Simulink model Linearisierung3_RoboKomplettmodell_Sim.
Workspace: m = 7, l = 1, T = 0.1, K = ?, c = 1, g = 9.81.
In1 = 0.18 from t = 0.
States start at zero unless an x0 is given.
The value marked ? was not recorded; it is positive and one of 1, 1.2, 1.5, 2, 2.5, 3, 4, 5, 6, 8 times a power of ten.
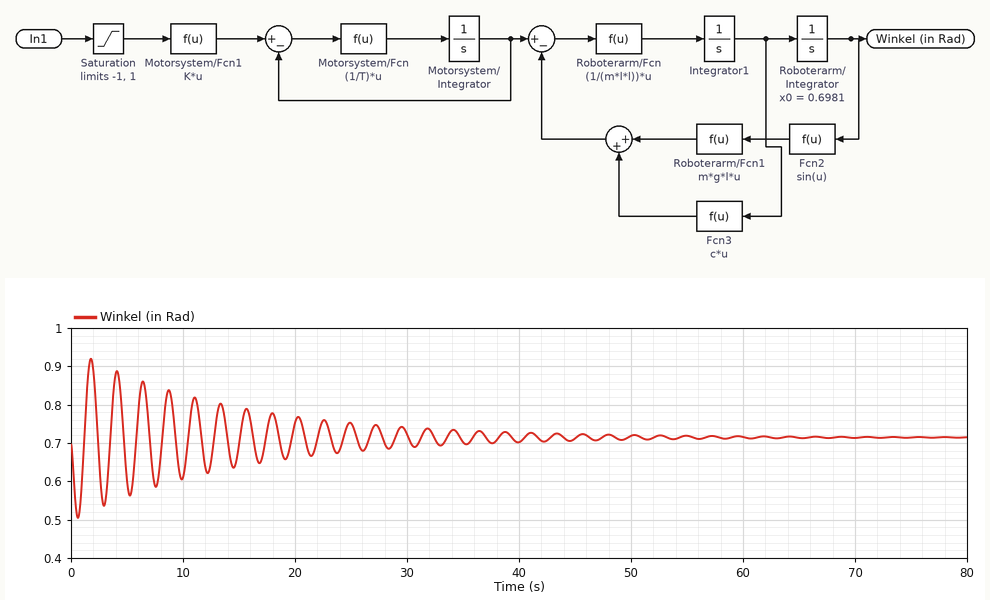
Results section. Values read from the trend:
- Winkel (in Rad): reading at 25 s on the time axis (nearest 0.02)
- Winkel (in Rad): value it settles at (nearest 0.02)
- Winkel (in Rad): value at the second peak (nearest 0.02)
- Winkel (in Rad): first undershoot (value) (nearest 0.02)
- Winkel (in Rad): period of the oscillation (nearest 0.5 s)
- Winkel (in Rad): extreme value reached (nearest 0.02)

0.76
0.72
0.88
0.54
2.5 s
0.92
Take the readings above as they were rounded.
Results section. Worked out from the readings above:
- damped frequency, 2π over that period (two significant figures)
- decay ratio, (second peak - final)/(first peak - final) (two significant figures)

2.5 rad/s
0.80
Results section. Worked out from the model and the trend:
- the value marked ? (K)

250
